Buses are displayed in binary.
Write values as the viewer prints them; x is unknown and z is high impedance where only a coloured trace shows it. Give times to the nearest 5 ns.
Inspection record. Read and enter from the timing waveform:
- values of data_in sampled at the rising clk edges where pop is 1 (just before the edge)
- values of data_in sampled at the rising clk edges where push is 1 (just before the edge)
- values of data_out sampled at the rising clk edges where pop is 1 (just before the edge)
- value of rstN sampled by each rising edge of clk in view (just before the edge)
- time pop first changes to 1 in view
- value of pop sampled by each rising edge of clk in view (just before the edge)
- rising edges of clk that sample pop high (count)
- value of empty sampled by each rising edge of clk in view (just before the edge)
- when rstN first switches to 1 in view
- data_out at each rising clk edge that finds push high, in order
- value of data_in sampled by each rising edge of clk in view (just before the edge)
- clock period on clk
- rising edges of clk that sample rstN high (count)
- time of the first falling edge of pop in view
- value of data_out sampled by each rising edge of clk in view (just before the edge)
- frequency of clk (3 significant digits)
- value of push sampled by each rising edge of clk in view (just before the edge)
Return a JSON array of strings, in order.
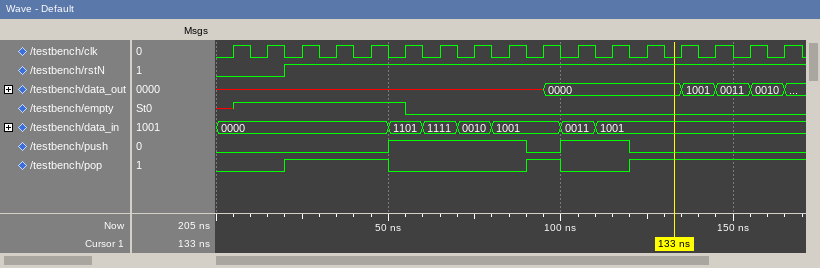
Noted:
["0000, 0000, 0000, 1001, 1001, 1001, 1001, 1001, 1001", "1101, 1111, 0010, 1001, 0011, 1001", "x, x, x, x, 0000, 0000, 1001, 0011, 0010", "0 0 1 1 1 1 1 1 1 1 1 1 1 1 1 1 1", "20 ns", "0 0 1 1 1 0 0 0 0 1 0 0 1 1 1 1 1", "9", "x 1 1 1 1 1 0 0 0 0 0 0 0 0 0 0 0", "20 ns", "x, x, x, x, 0000, 0000", "0000, 0000, 0000, 0000, 0000, 1101, 1111, 0010, 1001, 1001, 0011, 1001, 1001, 1001, 1001, 1001, 1001", "10 ns", "15", "50 ns", "x, x, x, x, x, x, x, x, x, x, 0000, 0000, 0000, 0000, 1001, 0011, 0010", "100 MHz", "0 0 0 0 0 1 1 1 1 0 1 1 0 0 0 0 0"]
